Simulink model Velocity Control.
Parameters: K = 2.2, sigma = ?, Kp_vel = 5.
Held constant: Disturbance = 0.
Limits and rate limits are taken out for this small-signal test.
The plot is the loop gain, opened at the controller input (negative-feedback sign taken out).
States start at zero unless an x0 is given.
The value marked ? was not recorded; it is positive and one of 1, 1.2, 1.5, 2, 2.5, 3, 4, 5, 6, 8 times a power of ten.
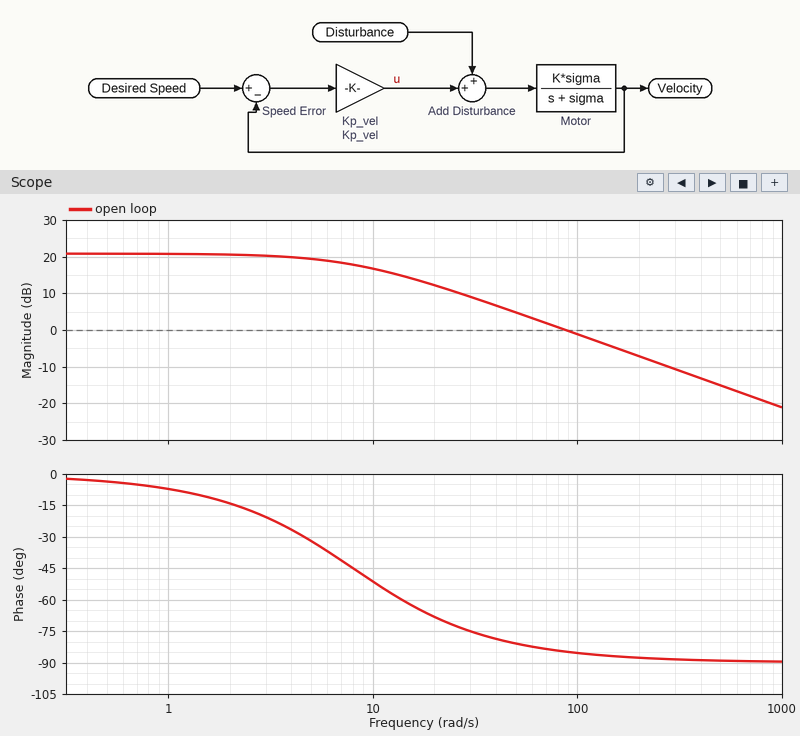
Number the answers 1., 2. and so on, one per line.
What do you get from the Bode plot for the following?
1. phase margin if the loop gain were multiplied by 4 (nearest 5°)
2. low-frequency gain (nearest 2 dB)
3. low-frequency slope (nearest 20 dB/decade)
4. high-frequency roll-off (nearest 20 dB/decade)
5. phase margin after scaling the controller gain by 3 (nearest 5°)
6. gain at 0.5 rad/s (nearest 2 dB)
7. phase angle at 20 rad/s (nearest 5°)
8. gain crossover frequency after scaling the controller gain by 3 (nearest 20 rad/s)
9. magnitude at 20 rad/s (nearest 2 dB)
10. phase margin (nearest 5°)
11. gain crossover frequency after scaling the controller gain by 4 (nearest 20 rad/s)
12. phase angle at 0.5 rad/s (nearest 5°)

1. 90°
2. 20 dB
3. 0 dB/decade
4. -20 dB/decade
5. 90°
6. 20 dB
7. -70°
8. 260 rad/s
9. 12 dB
10. 95°
11. 360 rad/s
12. -5°
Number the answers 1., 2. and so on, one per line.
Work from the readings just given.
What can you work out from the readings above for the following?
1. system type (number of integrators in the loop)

1. 0
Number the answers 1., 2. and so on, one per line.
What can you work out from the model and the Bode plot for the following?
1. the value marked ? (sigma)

1. 8
